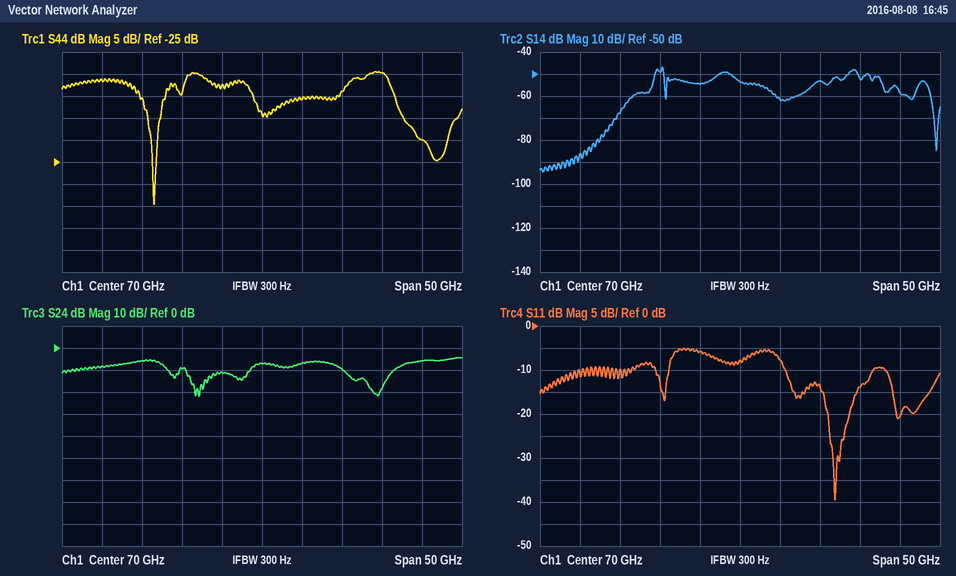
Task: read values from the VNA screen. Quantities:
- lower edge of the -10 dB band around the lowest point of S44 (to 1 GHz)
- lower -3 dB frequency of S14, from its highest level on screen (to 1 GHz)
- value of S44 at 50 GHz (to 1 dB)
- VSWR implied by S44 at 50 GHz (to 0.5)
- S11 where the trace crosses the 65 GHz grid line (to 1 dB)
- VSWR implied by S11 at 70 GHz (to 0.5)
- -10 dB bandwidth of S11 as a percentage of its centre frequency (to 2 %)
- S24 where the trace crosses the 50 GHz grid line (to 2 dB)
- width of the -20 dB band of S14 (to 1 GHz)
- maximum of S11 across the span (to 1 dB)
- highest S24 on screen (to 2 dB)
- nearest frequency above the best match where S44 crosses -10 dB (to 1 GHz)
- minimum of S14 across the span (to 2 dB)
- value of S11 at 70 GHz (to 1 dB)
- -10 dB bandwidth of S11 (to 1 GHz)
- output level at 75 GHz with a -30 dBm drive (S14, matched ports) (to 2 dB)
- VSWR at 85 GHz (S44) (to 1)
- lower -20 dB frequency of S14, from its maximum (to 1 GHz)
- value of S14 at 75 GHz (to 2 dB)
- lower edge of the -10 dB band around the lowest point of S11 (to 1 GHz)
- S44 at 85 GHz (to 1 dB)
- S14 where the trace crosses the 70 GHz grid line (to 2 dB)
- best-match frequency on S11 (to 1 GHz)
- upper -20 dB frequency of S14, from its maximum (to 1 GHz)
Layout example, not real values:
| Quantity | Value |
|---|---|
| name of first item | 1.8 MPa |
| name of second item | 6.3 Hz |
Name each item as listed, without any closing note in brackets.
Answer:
| Quantity | Value |
|---|---|
| lower edge of the -10 dB band around the lowest point of S44 | 55 GHz |
| lower -3 dB frequency of S14, from its highest level on screen | 59 GHz |
| value of S44 at 50 GHz | -6 dB |
| VSWR implied by S44 at 50 GHz | 3.0 |
| S11 where the trace crosses the 65 GHz grid line | -6 dB |
| VSWR implied by S11 at 70 GHz | 2.5 |
| -10 dB bandwidth of S11 as a percentage of its centre frequency | 14 % |
| S24 where the trace crosses the 50 GHz grid line | -8 dB |
| width of the -20 dB band of S14 | 39 GHz |
| maximum of S11 across the span | -5 dB |
| highest S24 on screen | -4 dB |
| nearest frequency above the best match where S44 crosses -10 dB | 58 GHz |
| minimum of S14 across the span | -94 dB |
| value of S11 at 70 GHz | -8 dB |
| -10 dB bandwidth of S11 | 11 GHz |
| output level at 75 GHz with a -30 dBm drive (S14, matched ports) | -92 dBm |
| VSWR at 85 GHz (S44) | 4 |
| lower -20 dB frequency of S14, from its maximum | 55 GHz |
| value of S14 at 75 GHz | -62 dB |
| lower edge of the -10 dB band around the lowest point of S11 | 76 GHz |
| S44 at 85 GHz | -5 dB |
| S14 where the trace crosses the 70 GHz grid line | -54 dB |
| best-match frequency on S11 | 82 GHz |
| upper -20 dB frequency of S14, from its maximum | 94 GHz |
